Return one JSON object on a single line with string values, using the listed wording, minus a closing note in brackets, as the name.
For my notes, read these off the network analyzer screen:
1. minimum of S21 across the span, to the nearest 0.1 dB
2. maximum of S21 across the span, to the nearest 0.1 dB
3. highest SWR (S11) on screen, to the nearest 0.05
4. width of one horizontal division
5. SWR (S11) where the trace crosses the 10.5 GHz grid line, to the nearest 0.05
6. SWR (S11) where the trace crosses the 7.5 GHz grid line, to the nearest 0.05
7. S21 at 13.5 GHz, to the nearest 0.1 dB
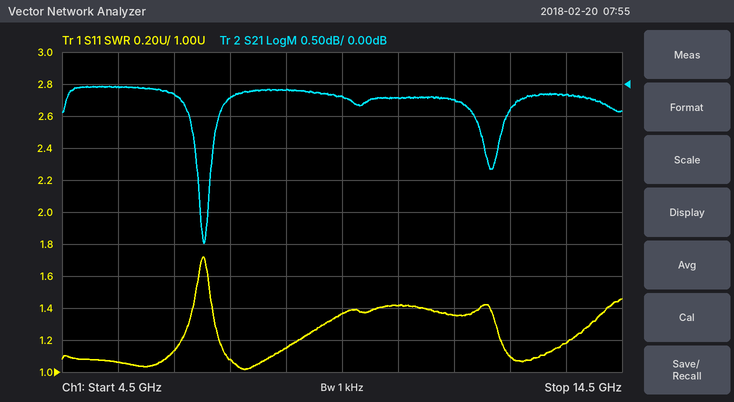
{"minimum of S21 across the span, to the nearest 0.1 dB": "-2.5 dB", "maximum of S21 across the span, to the nearest 0.1 dB": "0.0 dB", "highest SWR (S11) on screen, to the nearest 0.05": "1.70", "width of one horizontal division": "1 GHz", "SWR (S11) where the trace crosses the 10.5 GHz grid line, to the nearest 0.05": "1.40", "SWR (S11) where the trace crosses the 7.5 GHz grid line, to the nearest 0.05": "1.10", "S21 at 13.5 GHz, to the nearest 0.1 dB": "-0.2 dB"}
